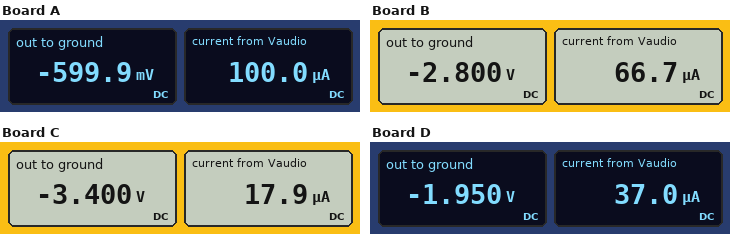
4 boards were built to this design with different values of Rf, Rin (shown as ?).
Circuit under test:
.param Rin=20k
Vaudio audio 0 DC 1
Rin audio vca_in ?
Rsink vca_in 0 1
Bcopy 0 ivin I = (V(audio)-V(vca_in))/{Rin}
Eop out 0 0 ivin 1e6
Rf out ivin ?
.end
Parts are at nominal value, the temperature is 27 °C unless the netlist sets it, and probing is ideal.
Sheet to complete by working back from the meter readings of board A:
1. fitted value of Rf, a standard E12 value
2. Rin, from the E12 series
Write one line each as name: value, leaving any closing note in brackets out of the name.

fitted value of Rf, a standard E12 value: 12 kΩ
Rin, from the E12 series: 10 kΩ
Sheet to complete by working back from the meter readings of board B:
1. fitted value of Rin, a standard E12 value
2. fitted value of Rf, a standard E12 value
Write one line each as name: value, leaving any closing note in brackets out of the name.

fitted value of Rin, a standard E12 value: 15 kΩ
fitted value of Rf, a standard E12 value: 56 kΩ
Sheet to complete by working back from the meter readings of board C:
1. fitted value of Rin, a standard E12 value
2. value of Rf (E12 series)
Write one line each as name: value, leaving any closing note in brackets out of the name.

fitted value of Rin, a standard E12 value: 56 kΩ
value of Rf: 68 kΩ
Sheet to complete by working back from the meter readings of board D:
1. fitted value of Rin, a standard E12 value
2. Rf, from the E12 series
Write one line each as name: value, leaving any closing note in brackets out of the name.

fitted value of Rin, a standard E12 value: 27 kΩ
Rf, from the E12 series: 39 kΩ
